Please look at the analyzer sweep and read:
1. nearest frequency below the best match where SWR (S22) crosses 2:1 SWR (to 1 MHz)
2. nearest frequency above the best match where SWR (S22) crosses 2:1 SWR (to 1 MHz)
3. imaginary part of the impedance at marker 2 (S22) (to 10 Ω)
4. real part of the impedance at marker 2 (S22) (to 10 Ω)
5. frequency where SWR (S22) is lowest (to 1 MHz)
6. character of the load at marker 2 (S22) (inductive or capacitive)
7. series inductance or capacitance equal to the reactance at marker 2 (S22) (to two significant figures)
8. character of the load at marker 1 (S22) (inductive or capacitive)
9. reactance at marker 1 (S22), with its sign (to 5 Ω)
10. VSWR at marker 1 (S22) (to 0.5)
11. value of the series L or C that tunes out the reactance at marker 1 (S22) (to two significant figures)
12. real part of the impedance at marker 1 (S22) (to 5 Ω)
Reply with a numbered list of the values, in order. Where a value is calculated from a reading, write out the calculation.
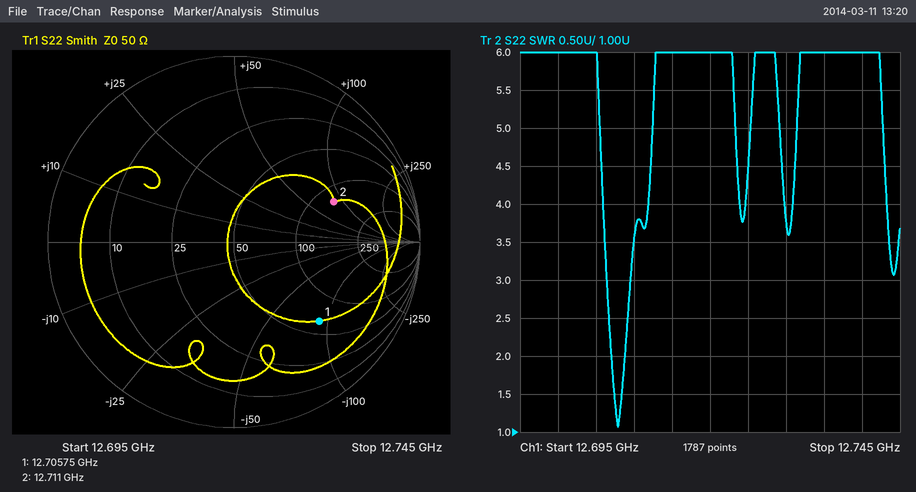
1. 12.707 GHz
2. 12.709 GHz
3. +80 Ω
4. 130 Ω
5. 12.708 GHz
6. inductive
7. L = 80 Ω/(2π × 12.711 GHz) ≈ 1.0 nH
8. capacitive
9. -90 Ω
10. 4.5
11. L = 90 Ω/(2π × 12.70575 GHz) ≈ 1.1 nH
12. 65 Ω
